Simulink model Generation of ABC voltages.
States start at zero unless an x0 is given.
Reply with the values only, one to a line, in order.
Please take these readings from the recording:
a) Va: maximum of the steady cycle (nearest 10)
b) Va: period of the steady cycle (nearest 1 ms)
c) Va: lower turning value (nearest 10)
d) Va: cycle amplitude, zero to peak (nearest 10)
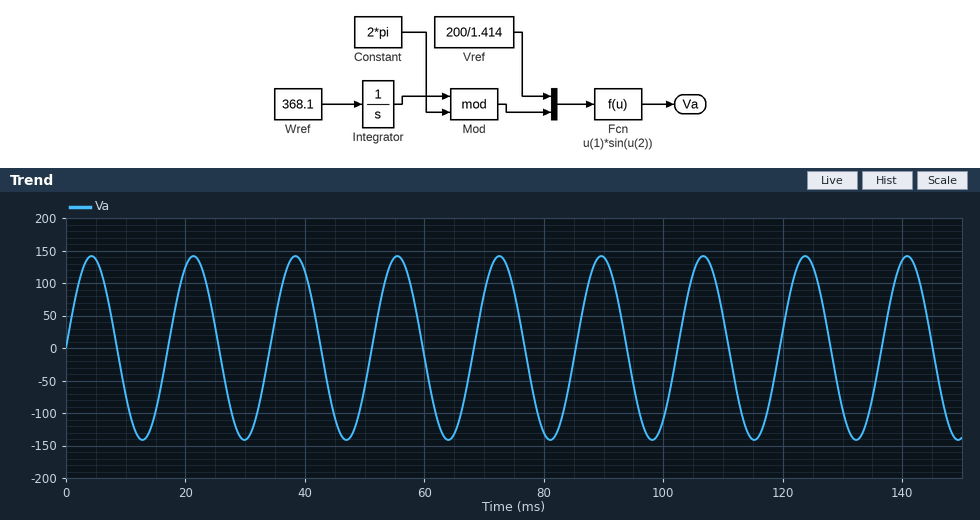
140
17 ms
-140
140
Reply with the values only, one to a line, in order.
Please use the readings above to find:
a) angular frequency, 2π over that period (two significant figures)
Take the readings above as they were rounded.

0.37 rad/ms
